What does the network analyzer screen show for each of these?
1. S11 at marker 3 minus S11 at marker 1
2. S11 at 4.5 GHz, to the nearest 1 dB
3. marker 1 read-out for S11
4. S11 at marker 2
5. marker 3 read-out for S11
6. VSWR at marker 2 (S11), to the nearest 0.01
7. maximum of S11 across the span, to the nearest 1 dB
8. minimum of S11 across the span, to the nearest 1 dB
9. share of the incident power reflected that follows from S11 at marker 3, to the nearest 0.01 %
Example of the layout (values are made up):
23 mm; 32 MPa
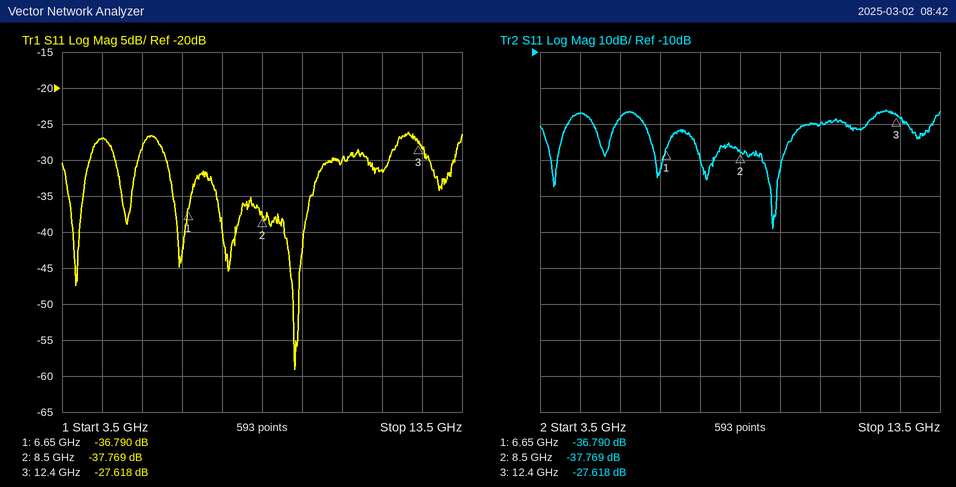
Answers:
9.172 dB; -27 dB; -36.790 dB; -37.769 dB; -27.618 dB; 1.03; -26 dB; -59 dB; 0.17 %
